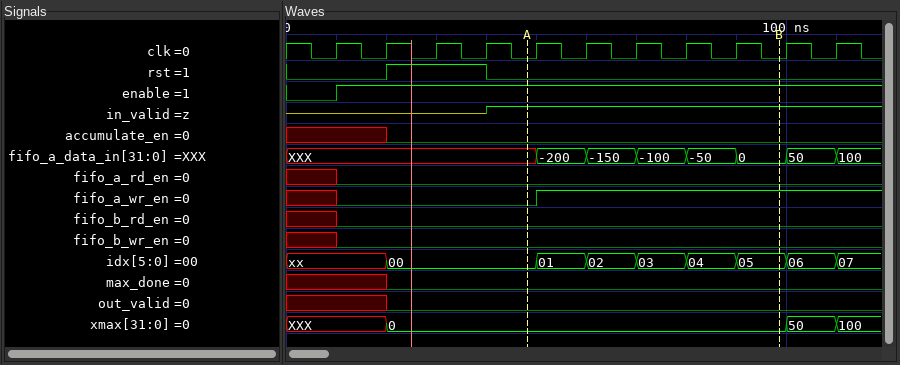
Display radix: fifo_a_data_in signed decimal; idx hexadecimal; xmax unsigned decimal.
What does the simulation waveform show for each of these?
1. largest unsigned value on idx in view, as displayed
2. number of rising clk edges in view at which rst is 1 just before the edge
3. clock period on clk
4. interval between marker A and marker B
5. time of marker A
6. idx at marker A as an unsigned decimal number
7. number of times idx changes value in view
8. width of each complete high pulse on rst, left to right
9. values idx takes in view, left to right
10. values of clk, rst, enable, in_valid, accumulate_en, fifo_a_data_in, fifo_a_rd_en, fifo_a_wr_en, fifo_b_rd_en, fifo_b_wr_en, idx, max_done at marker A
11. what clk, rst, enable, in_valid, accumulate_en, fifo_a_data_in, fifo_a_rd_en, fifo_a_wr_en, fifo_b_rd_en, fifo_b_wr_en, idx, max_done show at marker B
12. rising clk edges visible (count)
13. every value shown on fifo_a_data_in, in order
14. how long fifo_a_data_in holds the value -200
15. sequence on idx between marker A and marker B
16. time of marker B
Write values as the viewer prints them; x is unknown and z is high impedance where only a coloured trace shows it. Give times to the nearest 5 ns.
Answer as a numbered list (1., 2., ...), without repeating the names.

1. 07
2. 2
3. 10 ns
4. 50 ns
5. 50 ns
6. 0
7. 8
8. 20 ns
9. xx, 00, 01, 02, 03, 04, 05, 06, 07
10. clk=0, rst=0, enable=1, in_valid=1, accumulate_en=0, fifo_a_data_in=XXX, fifo_a_rd_en=0, fifo_a_wr_en=0, fifo_b_rd_en=0, fifo_b_wr_en=0, idx=00, max_done=0
11. clk=0, rst=0, enable=1, in_valid=1, accumulate_en=0, fifo_a_data_in=0, fifo_a_rd_en=0, fifo_a_wr_en=1, fifo_b_rd_en=0, fifo_b_wr_en=0, idx=05, max_done=0
12. 11
13. XXX, -200, -150, -100, -50, 0, 50, 100
14. 10 ns
15. 00, 01, 02, 03, 04, 05
16. 100 ns
